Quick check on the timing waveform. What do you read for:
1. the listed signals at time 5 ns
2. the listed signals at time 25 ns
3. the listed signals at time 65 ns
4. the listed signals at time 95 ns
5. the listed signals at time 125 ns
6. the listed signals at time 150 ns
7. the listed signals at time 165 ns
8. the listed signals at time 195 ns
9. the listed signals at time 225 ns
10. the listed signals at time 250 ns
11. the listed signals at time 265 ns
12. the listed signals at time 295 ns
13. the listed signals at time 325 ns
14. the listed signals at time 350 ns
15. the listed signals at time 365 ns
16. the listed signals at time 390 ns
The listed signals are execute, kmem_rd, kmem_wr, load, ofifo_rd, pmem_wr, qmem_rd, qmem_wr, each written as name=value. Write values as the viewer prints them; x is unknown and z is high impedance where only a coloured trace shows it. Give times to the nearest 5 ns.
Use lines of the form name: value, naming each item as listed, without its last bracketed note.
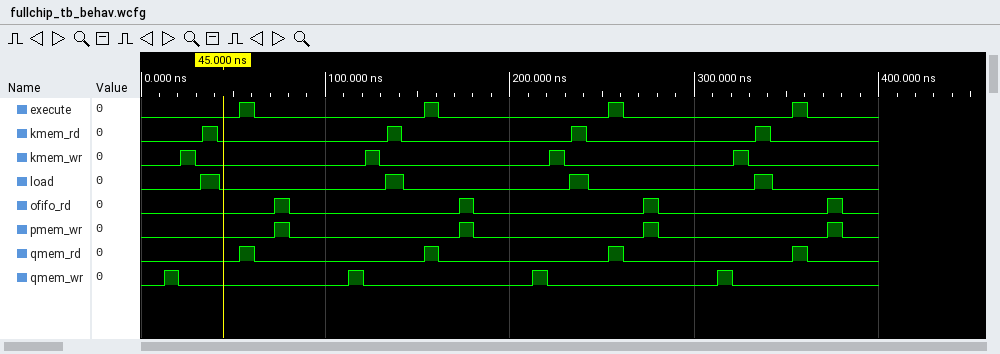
the listed signals at time 5 ns: execute=0, kmem_rd=0, kmem_wr=0, load=0, ofifo_rd=0, pmem_wr=0, qmem_rd=0, qmem_wr=0
the listed signals at time 25 ns: execute=0, kmem_rd=0, kmem_wr=1, load=0, ofifo_rd=0, pmem_wr=0, qmem_rd=0, qmem_wr=0
the listed signals at time 65 ns: execute=0, kmem_rd=0, kmem_wr=0, load=0, ofifo_rd=0, pmem_wr=0, qmem_rd=0, qmem_wr=0
the listed signals at time 95 ns: execute=0, kmem_rd=0, kmem_wr=0, load=0, ofifo_rd=0, pmem_wr=0, qmem_rd=0, qmem_wr=0
the listed signals at time 125 ns: execute=0, kmem_rd=0, kmem_wr=1, load=0, ofifo_rd=0, pmem_wr=0, qmem_rd=0, qmem_wr=0
the listed signals at time 150 ns: execute=0, kmem_rd=0, kmem_wr=0, load=0, ofifo_rd=0, pmem_wr=0, qmem_rd=0, qmem_wr=0
the listed signals at time 165 ns: execute=0, kmem_rd=0, kmem_wr=0, load=0, ofifo_rd=0, pmem_wr=0, qmem_rd=0, qmem_wr=0
the listed signals at time 195 ns: execute=0, kmem_rd=0, kmem_wr=0, load=0, ofifo_rd=0, pmem_wr=0, qmem_rd=0, qmem_wr=0
the listed signals at time 225 ns: execute=0, kmem_rd=0, kmem_wr=1, load=0, ofifo_rd=0, pmem_wr=0, qmem_rd=0, qmem_wr=0
the listed signals at time 250 ns: execute=0, kmem_rd=0, kmem_wr=0, load=0, ofifo_rd=0, pmem_wr=0, qmem_rd=0, qmem_wr=0
the listed signals at time 265 ns: execute=0, kmem_rd=0, kmem_wr=0, load=0, ofifo_rd=0, pmem_wr=0, qmem_rd=0, qmem_wr=0
the listed signals at time 295 ns: execute=0, kmem_rd=0, kmem_wr=0, load=0, ofifo_rd=0, pmem_wr=0, qmem_rd=0, qmem_wr=0
the listed signals at time 325 ns: execute=0, kmem_rd=0, kmem_wr=1, load=0, ofifo_rd=0, pmem_wr=0, qmem_rd=0, qmem_wr=0
the listed signals at time 350 ns: execute=0, kmem_rd=0, kmem_wr=0, load=0, ofifo_rd=0, pmem_wr=0, qmem_rd=0, qmem_wr=0
the listed signals at time 365 ns: execute=0, kmem_rd=0, kmem_wr=0, load=0, ofifo_rd=0, pmem_wr=0, qmem_rd=0, qmem_wr=0
the listed signals at time 390 ns: execute=0, kmem_rd=0, kmem_wr=0, load=0, ofifo_rd=0, pmem_wr=0, qmem_rd=0, qmem_wr=0
